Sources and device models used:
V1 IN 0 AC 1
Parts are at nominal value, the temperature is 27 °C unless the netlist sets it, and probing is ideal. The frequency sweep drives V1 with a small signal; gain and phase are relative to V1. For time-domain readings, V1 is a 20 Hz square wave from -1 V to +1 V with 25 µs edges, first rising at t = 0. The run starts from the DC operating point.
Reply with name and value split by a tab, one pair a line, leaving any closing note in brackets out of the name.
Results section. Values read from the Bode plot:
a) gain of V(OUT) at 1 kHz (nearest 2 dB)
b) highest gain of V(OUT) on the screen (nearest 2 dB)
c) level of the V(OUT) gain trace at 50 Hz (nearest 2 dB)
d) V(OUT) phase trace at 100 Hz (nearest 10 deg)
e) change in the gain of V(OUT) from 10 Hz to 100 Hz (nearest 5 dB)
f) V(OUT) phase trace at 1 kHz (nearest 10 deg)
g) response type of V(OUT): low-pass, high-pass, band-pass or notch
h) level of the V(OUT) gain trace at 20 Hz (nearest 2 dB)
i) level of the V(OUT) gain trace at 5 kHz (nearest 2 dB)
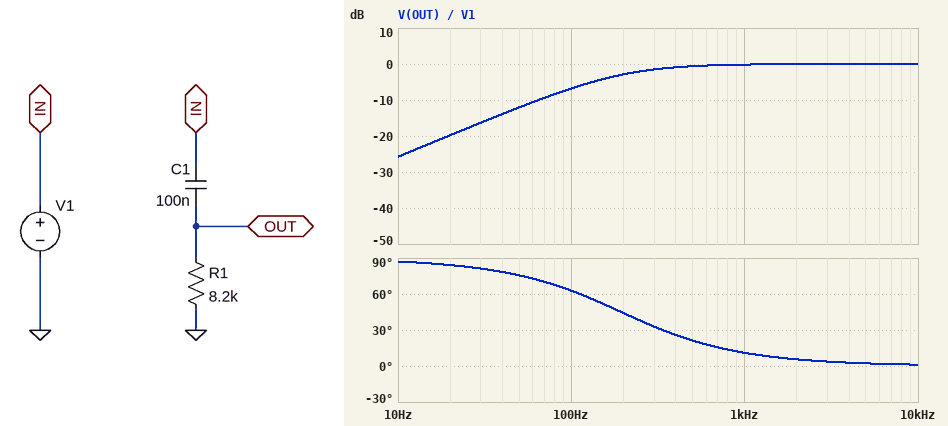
gain of V(OUT) at 1 kHz	0 dB
highest gain of V(OUT) on the screen	0 dB
level of the V(OUT) gain trace at 50 Hz	-12 dB
V(OUT) phase trace at 100 Hz	60 deg
change in the gain of V(OUT) from 10 Hz to 100 Hz	20 dB
V(OUT) phase trace at 1 kHz	10 deg
response type of V(OUT): low-pass, high-pass, band-pass or notch	high-pass
level of the V(OUT) gain trace at 20 Hz	-20 dB
level of the V(OUT) gain trace at 5 kHz	0 dB
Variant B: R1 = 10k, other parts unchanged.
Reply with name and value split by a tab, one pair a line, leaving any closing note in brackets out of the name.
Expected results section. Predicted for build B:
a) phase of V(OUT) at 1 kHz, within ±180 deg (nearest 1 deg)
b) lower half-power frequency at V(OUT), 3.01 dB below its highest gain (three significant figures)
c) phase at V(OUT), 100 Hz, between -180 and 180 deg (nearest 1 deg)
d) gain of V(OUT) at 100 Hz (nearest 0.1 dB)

phase of V(OUT) at 1 kHz, within ±180 deg	9 deg
lower half-power frequency at V(OUT), 3.01 dB below its highest gain	159 Hz
phase at V(OUT), 100 Hz, between -180 and 180 deg	58 deg
gain of V(OUT) at 100 Hz	-5.5 dB
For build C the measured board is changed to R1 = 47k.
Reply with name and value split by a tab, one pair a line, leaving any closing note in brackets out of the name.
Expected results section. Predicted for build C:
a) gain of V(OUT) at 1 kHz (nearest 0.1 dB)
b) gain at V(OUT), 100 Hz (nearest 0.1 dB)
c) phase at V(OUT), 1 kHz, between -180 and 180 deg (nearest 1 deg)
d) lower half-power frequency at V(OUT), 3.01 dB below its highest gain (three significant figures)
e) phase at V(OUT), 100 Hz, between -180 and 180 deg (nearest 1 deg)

gain of V(OUT) at 1 kHz	0 dB
gain at V(OUT), 100 Hz	-0.5 dB
phase at V(OUT), 1 kHz, between -180 and 180 deg	2 deg
lower half-power frequency at V(OUT), 3.01 dB below its highest gain	33.9 Hz
phase at V(OUT), 100 Hz, between -180 and 180 deg	19 deg
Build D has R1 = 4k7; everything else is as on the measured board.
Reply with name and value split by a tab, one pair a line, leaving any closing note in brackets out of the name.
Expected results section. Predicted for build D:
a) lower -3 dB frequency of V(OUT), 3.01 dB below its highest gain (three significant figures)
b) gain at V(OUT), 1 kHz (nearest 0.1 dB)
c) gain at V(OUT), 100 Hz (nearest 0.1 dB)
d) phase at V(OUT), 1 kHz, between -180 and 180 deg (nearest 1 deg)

lower -3 dB frequency of V(OUT), 3.01 dB below its highest gain	339 Hz
gain at V(OUT), 1 kHz	-0.5 dB
gain at V(OUT), 100 Hz	-11.0 dB
phase at V(OUT), 1 kHz, between -180 and 180 deg	19 deg
